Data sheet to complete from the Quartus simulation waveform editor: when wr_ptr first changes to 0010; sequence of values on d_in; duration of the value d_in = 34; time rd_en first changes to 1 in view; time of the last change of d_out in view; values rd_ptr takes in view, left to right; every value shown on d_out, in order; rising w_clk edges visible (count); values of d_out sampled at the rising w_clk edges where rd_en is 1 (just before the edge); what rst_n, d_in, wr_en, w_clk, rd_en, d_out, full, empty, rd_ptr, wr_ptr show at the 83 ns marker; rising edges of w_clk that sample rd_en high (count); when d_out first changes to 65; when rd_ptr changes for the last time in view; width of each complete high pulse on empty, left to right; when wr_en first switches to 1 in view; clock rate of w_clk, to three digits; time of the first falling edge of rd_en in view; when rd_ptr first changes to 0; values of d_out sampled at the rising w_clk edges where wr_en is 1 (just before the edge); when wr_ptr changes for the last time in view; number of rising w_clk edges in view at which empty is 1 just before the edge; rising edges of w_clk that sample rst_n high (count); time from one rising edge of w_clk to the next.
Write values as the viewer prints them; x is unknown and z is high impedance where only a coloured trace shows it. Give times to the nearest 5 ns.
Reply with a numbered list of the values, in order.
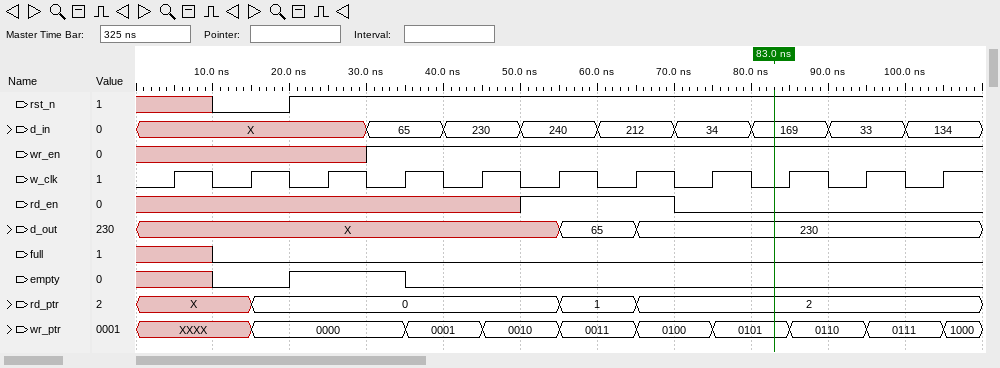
1. 45 ns
2. X, 65, 230, 240, 212, 34, 169, 33, 134
3. 10 ns
4. 50 ns
5. 65 ns
6. X, 0, 1, 2
7. X, 65, 230
8. 11
9. X, 65
10. rst_n=1, d_in=169, wr_en=1, w_clk=0, rd_en=0, d_out=230, full=0, empty=0, rd_ptr=2, wr_ptr=0101
11. 2
12. 55 ns
13. 65 ns
14. 15 ns
15. 30 ns
16. 100 MHz
17. 70 ns
18. 15 ns
19. X, X, X, 65, 230, 230, 230, 230
20. 105 ns
21. 2
22. 9
23. 10 ns
